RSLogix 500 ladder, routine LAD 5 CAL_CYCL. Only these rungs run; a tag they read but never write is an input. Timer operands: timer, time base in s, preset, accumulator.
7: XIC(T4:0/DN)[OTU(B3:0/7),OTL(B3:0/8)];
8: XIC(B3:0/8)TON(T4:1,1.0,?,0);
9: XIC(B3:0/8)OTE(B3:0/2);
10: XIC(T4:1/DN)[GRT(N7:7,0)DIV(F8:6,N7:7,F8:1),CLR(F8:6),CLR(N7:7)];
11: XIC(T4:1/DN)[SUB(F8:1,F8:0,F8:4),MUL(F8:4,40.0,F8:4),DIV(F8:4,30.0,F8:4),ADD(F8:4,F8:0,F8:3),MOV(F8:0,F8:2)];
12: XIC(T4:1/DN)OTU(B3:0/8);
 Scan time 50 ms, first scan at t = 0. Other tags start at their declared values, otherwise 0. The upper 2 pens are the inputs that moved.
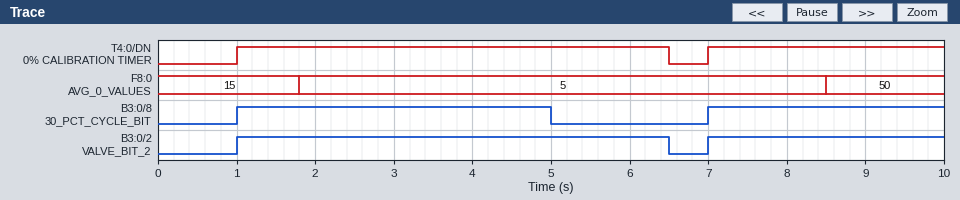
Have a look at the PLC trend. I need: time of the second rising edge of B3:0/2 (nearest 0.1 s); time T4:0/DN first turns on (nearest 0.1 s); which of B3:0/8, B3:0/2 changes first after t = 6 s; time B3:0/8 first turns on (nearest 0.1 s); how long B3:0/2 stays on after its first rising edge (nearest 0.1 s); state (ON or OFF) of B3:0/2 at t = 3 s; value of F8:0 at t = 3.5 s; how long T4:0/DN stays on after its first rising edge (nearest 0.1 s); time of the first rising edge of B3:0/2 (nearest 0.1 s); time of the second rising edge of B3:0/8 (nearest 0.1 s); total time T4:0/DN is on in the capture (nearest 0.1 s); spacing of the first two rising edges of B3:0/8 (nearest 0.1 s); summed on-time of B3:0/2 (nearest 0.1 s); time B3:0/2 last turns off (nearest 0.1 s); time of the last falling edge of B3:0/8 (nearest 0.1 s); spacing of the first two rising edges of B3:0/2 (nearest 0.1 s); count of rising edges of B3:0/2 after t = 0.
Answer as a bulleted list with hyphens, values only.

- 7.0 s
- 1.0 s
- B3:0/2
- 1.0 s
- 5.5 s
- ON
- 5
- 5.5 s
- 1.0 s
- 7.0 s
- 8.5 s
- 6.0 s
- 8.5 s
- 6.5 s
- 5.0 s
- 6.0 s
- 2
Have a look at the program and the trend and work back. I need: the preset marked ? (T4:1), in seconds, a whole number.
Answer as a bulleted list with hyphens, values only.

- 4 s
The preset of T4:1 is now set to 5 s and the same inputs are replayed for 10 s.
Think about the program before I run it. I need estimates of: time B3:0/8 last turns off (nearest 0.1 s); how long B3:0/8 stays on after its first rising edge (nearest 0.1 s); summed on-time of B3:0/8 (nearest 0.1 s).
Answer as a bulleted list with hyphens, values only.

- 6.0 s
- 5.0 s
- 8.0 s
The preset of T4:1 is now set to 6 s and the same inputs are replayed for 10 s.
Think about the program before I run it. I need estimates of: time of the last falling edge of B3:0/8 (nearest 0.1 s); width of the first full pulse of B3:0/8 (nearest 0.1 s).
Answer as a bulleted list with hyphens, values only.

- 7.0 s
- 6.0 s
